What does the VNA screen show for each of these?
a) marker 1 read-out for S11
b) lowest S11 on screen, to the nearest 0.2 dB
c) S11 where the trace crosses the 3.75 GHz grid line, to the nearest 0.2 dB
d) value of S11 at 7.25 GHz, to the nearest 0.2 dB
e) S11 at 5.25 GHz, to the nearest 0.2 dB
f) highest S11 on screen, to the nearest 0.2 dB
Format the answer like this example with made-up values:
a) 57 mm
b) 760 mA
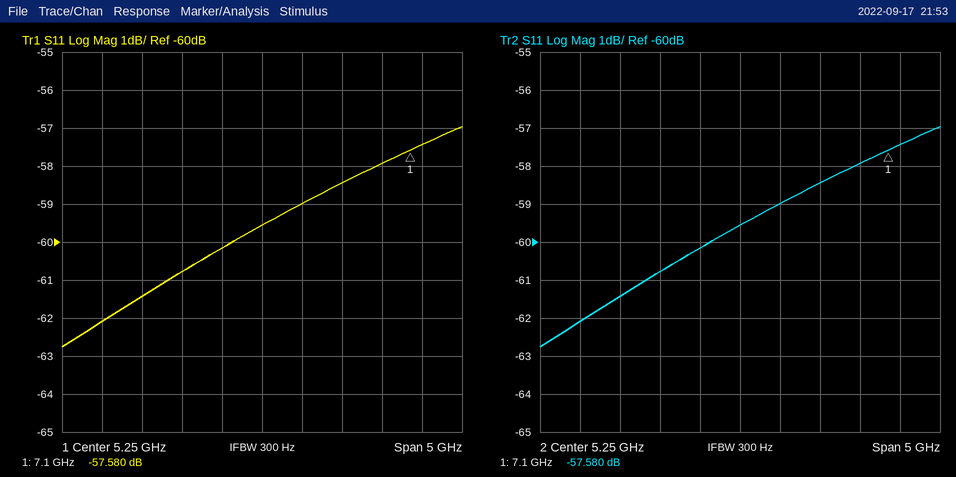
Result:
a) -57.580 dB
b) -62.8 dB
c) -61.4 dB
d) -57.4 dB
e) -59.6 dB
f) -57.0 dB
